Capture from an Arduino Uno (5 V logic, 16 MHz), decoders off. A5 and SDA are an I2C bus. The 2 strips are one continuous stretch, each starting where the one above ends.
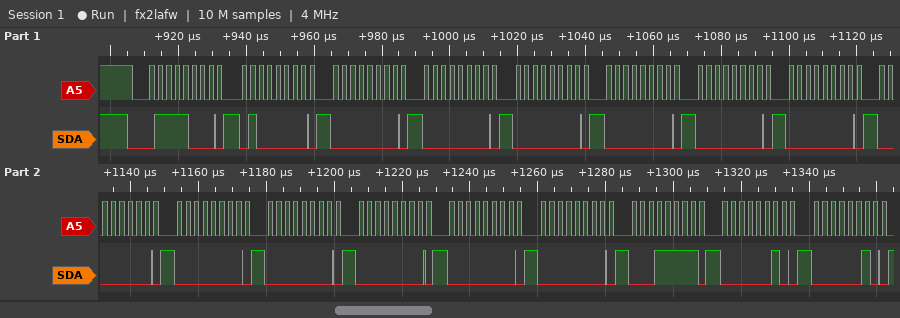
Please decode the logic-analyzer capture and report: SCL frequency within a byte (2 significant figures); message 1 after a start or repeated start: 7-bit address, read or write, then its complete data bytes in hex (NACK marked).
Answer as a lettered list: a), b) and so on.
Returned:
a) 400 kHz
b) 0x3C write: 40 00 00 00 00 00 00 00 00 00 00 00 00 1F 02 02
